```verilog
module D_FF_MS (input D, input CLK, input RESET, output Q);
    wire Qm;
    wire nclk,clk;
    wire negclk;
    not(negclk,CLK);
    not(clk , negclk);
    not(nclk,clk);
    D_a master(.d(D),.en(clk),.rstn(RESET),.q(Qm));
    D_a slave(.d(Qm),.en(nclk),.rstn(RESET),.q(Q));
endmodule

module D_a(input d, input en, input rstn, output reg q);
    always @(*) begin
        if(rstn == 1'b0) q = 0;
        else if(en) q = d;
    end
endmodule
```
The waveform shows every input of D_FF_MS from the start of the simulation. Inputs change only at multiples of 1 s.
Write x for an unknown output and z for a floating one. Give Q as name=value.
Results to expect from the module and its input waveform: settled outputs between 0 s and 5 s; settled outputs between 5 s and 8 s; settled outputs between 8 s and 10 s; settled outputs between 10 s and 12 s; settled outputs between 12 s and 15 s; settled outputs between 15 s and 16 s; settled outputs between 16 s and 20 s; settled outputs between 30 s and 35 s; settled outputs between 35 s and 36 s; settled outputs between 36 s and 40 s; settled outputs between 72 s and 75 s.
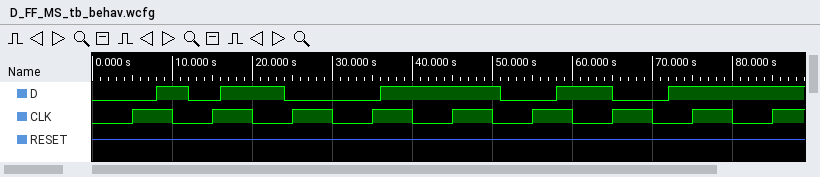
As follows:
Q=x
Q=x
Q=x
Q=1
Q=1
Q=1
Q=1
Q=0
Q=0
Q=0
Q=0
